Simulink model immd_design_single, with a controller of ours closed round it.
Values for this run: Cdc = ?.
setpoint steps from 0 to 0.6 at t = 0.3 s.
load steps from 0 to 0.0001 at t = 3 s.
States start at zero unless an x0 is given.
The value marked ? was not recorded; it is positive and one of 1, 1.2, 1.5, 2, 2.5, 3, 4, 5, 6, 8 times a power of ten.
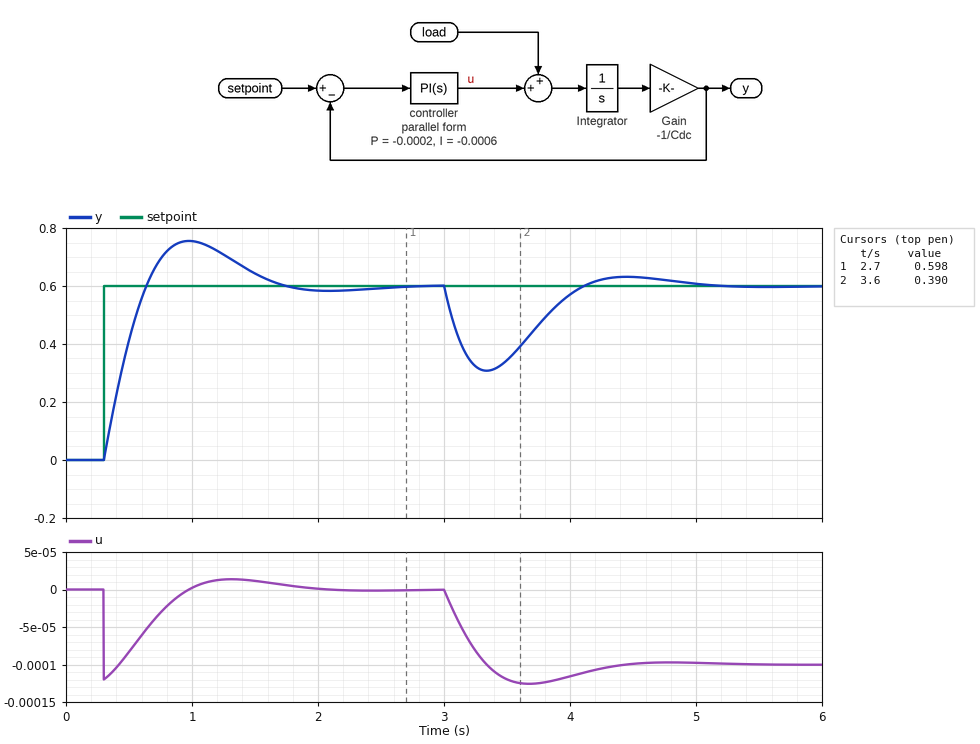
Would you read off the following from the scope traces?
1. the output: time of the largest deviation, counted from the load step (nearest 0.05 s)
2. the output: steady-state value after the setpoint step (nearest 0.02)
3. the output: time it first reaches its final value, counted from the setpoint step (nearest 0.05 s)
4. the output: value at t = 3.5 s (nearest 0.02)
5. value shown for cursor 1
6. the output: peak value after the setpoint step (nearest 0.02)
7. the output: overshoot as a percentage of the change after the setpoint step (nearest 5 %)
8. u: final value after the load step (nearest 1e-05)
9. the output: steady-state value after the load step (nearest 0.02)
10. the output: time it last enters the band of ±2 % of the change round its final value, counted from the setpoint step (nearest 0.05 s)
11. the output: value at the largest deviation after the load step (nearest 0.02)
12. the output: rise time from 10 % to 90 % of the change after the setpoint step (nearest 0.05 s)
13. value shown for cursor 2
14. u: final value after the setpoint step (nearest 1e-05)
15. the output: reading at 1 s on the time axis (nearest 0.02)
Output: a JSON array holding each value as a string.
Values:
["0.35 s", "0.60", "0.35 s", "0.34", "0.598", "0.76", "25 %", "-0.00010", "0.60", "2.05 s", "0.30", "0.25 s", "0.390", "0.00000", "0.76"]
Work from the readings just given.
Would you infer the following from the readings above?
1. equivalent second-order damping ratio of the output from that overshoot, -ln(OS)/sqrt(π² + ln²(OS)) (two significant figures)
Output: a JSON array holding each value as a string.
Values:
["0.40"]
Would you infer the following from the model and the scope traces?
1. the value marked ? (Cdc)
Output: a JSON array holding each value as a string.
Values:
["5e-05"]
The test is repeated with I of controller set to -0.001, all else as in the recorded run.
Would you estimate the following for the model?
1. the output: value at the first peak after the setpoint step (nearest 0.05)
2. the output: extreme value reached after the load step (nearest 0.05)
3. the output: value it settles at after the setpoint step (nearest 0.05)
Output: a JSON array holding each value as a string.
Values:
["0.80", "0.35", "0.60"]
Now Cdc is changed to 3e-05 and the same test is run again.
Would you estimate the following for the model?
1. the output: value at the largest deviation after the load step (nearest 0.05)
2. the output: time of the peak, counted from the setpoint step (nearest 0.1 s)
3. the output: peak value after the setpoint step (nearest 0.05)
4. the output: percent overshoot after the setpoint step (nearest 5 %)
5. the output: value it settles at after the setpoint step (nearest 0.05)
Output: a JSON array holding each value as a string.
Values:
["0.25", "0.5 s", "0.70", "20 %", "0.60"]
